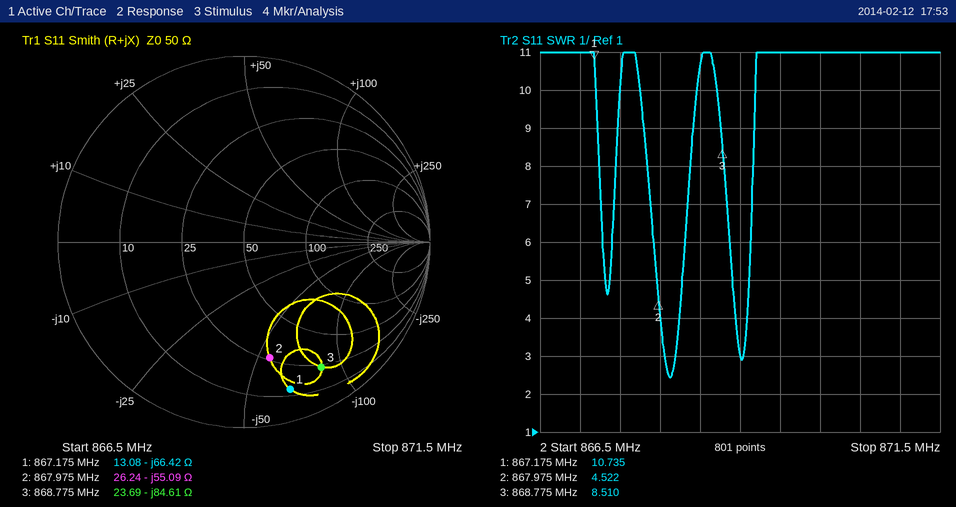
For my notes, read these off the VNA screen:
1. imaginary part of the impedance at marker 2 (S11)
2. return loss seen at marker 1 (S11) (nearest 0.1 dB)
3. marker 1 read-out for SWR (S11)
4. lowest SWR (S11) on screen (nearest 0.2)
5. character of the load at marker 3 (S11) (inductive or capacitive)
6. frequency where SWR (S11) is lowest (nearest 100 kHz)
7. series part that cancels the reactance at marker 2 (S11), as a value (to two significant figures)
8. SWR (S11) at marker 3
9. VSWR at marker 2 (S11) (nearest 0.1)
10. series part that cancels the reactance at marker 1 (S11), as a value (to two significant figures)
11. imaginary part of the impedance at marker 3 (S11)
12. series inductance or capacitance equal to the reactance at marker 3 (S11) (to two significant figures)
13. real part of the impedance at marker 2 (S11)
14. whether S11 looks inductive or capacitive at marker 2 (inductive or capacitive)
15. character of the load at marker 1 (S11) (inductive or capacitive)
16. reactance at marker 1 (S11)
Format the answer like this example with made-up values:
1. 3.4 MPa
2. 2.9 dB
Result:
1. -55.09 Ω
2. 1.6 dB
3. 10.735
4. 2.4
5. capacitive
6. 868.1 MHz
7. 10 nH
8. 8.510
9. 4.5
10. 12 nH
11. -84.61 Ω
12. 2.2 pF
13. 26.24 Ω
14. capacitive
15. capacitive
16. -66.42 Ω
